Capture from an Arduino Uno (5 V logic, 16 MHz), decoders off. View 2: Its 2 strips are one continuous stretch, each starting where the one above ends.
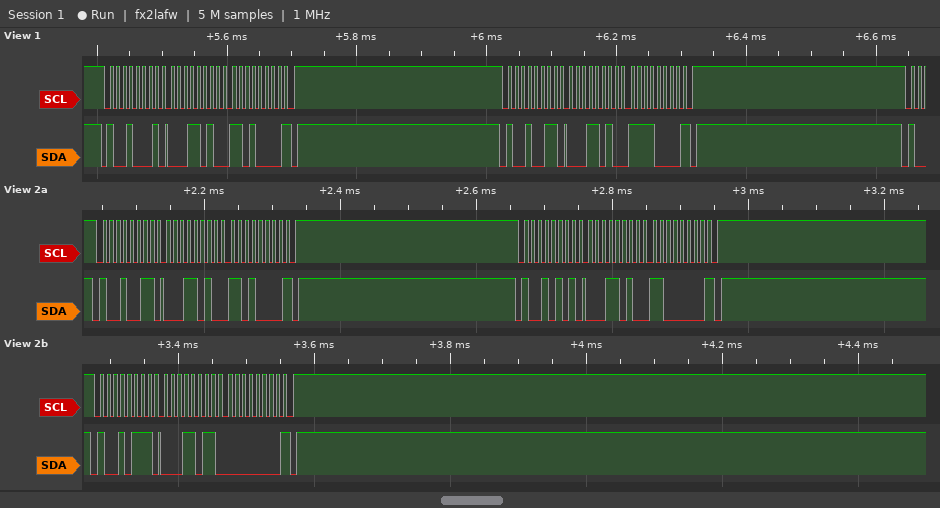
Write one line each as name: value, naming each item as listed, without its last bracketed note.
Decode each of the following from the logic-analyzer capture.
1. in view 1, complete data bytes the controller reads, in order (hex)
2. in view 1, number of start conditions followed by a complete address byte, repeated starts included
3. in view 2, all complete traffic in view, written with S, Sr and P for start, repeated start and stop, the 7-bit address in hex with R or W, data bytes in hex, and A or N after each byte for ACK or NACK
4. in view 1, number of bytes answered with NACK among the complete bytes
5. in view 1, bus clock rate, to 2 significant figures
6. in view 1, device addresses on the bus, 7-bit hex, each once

in view 1, complete data bytes the controller reads, in order: 1A D0 1A F0
in view 1, number of start conditions followed by a complete address byte, repeated starts included: 2
in view 2, all complete traffic in view, written with S, Sr and P for start, repeated start and stop, the 7-bit address in hex with R or W, data bytes in hex, and A or N after each byte for ACK or NACK: S 49R A 1A A D0 N P S 4AR A 1A A C0 N P S 4BR A 1B A 00 N P
in view 1, number of bytes answered with NACK among the complete bytes: 2
in view 1, bus clock rate, to 2 significant figures: 100 kHz
in view 1, device addresses on the bus, 7-bit hex, each once: 0x48 0x49
